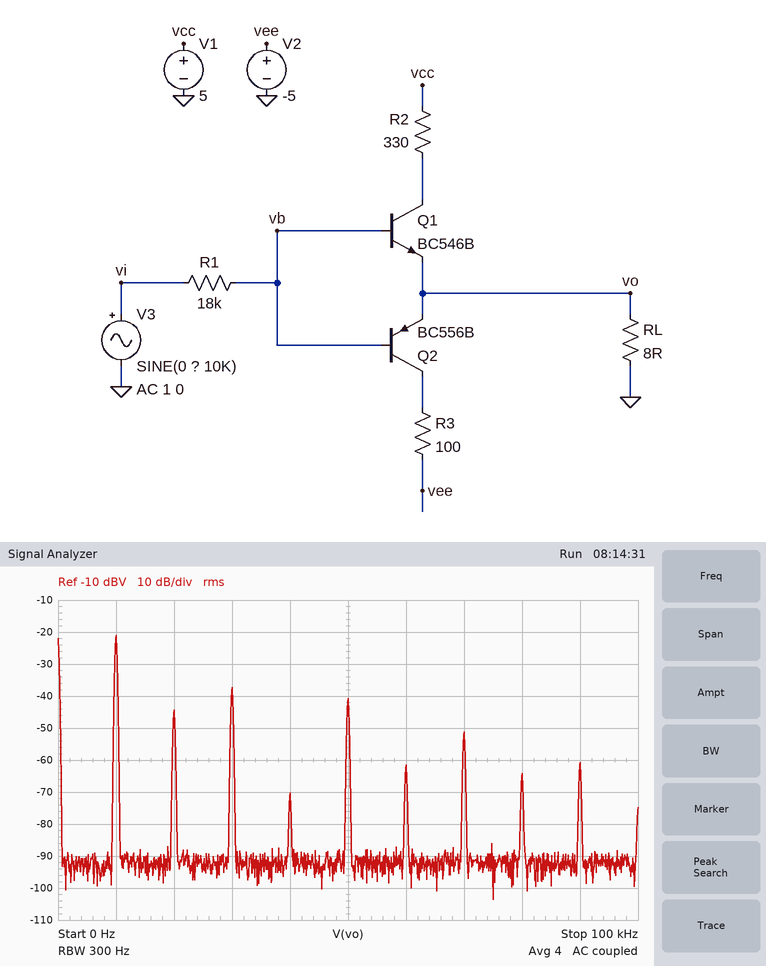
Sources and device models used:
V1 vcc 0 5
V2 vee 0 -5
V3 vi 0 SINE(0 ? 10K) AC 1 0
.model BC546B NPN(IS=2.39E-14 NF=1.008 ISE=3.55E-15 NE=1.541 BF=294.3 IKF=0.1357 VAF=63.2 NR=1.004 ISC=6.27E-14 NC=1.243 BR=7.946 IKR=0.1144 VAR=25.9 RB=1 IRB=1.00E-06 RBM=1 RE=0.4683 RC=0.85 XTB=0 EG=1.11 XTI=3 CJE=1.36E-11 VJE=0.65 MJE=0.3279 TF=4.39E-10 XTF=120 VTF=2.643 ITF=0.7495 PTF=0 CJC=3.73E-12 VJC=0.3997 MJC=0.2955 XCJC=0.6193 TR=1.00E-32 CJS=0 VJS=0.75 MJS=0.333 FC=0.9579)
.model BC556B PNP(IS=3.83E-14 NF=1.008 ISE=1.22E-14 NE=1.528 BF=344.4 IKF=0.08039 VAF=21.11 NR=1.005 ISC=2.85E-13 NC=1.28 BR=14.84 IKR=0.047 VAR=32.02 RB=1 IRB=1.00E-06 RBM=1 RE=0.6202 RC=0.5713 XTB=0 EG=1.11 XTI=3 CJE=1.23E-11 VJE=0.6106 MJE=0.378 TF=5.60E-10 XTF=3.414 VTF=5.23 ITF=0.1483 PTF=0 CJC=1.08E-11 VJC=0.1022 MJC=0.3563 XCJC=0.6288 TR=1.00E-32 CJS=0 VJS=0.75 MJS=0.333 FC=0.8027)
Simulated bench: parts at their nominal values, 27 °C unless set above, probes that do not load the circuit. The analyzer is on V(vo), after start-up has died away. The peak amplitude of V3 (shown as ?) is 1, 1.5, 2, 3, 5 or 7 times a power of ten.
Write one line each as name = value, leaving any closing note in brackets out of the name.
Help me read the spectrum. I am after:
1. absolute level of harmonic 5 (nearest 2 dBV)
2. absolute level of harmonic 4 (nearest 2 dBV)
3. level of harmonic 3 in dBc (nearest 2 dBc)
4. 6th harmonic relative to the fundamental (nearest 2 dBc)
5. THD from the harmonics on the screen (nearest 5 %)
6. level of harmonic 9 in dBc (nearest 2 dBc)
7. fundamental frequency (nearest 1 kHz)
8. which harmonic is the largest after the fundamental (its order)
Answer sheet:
absolute level of harmonic 5 = -40 dBV
absolute level of harmonic 4 = -70 dBV
level of harmonic 3 in dBc = -16 dBc
6th harmonic relative to the fundamental = -40 dBc
THD from the harmonics on the screen = 20 %
level of harmonic 9 in dBc = -40 dBc
fundamental frequency = 10 kHz
which harmonic is the largest after the fundamental = 3
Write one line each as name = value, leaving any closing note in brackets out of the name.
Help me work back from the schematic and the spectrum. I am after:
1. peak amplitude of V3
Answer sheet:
peak amplitude of V3 = 2 V
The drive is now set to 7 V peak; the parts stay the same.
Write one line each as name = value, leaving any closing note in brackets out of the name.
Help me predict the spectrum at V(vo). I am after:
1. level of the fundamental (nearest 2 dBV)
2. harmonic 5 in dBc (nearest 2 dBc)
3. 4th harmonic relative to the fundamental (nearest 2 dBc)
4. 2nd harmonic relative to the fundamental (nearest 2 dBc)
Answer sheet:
level of the fundamental = -14 dBV
harmonic 5 in dBc = -36 dBc
4th harmonic relative to the fundamental = -20 dBc
2nd harmonic relative to the fundamental = -14 dBc
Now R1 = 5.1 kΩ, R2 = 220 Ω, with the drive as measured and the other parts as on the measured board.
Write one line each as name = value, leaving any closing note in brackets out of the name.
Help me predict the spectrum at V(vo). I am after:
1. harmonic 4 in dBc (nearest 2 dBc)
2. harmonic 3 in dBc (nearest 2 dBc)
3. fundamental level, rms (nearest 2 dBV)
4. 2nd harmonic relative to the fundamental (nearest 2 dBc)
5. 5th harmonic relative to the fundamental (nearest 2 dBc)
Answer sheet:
harmonic 4 in dBc = -30 dBc
harmonic 3 in dBc = -20 dBc
fundamental level, rms = -16 dBV
2nd harmonic relative to the fundamental = -16 dBc
5th harmonic relative to the fundamental = -18 dBc
